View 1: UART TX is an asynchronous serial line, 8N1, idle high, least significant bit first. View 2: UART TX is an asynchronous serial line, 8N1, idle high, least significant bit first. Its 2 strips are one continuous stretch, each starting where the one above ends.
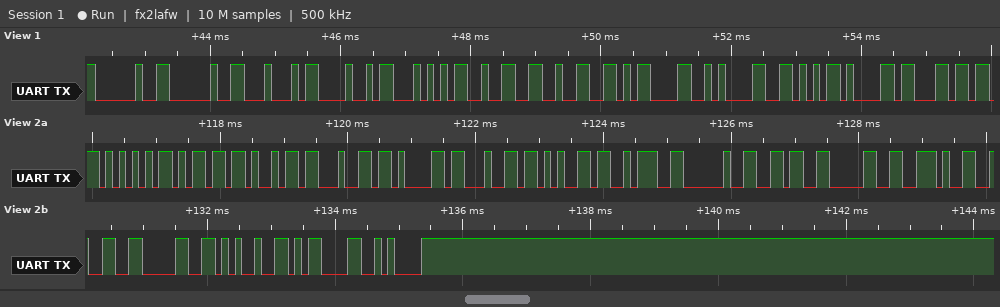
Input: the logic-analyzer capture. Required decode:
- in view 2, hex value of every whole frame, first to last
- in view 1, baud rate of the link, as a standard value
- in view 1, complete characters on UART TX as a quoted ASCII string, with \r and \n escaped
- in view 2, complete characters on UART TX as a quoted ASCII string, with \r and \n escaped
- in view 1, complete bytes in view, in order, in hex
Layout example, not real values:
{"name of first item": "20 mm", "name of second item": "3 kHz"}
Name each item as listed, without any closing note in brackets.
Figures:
{"in view 2, hex value of every whole frame, first to last": "55 6D 69 64 61 64 65 3A 20 36 30 2E 32 30 25 0D 0A", "in view 1, baud rate of the link, as a standard value": "9600 baud", "in view 1, complete characters on UART TX as a quoted ASCII string, with \\r and \\n escaped": "\"  DHT22\\r\\nVal\"", "in view 2, complete characters on UART TX as a quoted ASCII string, with \\r and \\n escaped": "\"Umidade: 60.20%\\r\\n\"", "in view 1, complete bytes in view, in order, in hex": "0x20 0x20 0x44 0x48 0x54 0x32 0x32 0x0D 0x0A 0x56 0x61 0x6C"}
